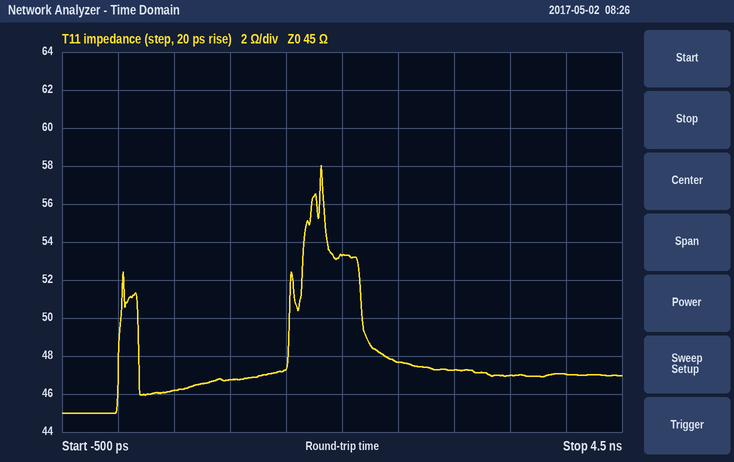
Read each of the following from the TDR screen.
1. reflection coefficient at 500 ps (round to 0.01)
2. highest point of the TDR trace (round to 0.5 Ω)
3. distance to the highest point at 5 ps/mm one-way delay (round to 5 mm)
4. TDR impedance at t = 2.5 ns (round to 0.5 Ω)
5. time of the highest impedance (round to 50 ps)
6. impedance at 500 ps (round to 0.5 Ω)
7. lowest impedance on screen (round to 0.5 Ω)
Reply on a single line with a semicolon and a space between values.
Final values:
+0.01; 58.0 Ω; 180 mm; 47.5 Ω; 1.80 ns; 46.0 Ω; 45.0 Ω
